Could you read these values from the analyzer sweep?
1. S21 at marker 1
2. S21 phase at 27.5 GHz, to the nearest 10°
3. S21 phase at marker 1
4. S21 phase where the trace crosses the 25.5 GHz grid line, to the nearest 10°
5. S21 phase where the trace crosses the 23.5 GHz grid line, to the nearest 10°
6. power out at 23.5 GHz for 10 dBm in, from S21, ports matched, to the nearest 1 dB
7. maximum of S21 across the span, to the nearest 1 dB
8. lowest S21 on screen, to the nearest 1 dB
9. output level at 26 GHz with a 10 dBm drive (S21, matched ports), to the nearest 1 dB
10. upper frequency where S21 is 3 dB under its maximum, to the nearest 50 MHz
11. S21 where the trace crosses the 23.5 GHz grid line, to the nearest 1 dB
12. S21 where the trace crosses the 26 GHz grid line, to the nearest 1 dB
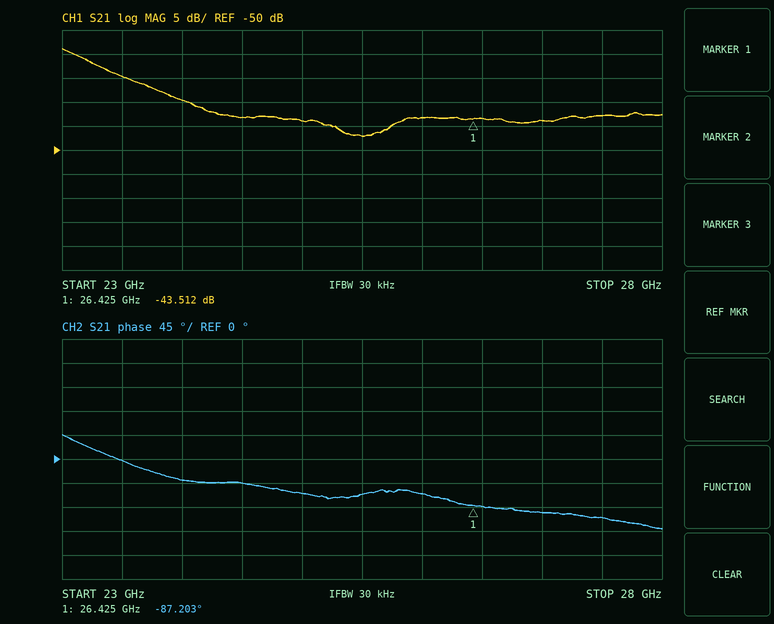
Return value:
-43.512 dB
-110°
-87.203°
-70°
0°
-25 dBm
-29 dB
-47 dB
-33 dBm
23.25 GHz
-35 dB
-43 dB
